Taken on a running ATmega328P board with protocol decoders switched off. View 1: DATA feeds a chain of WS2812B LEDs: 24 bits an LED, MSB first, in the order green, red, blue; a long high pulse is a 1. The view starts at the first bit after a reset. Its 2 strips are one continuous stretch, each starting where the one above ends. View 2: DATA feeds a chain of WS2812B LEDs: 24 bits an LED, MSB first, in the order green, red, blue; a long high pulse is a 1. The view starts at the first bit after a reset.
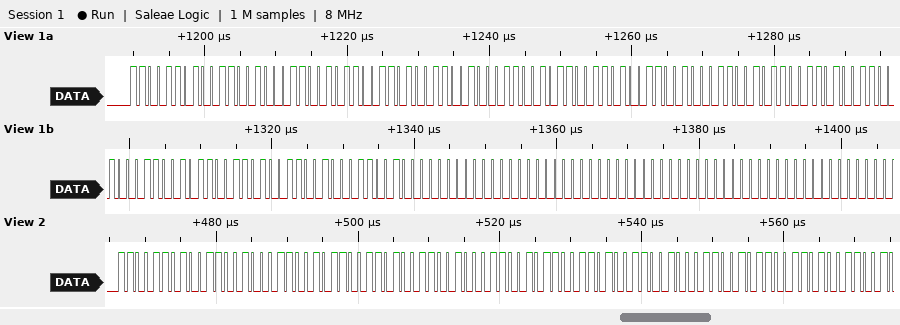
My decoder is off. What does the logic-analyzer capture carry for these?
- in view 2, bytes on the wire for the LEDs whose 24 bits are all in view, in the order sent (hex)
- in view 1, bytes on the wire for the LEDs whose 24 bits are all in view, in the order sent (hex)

CD 32 32 CD 32 32 CD 32 32
CD 32 32 CD 32 32 CD 32 32 CD 32 32 CD 32 32 00 00 00 00 00 00
